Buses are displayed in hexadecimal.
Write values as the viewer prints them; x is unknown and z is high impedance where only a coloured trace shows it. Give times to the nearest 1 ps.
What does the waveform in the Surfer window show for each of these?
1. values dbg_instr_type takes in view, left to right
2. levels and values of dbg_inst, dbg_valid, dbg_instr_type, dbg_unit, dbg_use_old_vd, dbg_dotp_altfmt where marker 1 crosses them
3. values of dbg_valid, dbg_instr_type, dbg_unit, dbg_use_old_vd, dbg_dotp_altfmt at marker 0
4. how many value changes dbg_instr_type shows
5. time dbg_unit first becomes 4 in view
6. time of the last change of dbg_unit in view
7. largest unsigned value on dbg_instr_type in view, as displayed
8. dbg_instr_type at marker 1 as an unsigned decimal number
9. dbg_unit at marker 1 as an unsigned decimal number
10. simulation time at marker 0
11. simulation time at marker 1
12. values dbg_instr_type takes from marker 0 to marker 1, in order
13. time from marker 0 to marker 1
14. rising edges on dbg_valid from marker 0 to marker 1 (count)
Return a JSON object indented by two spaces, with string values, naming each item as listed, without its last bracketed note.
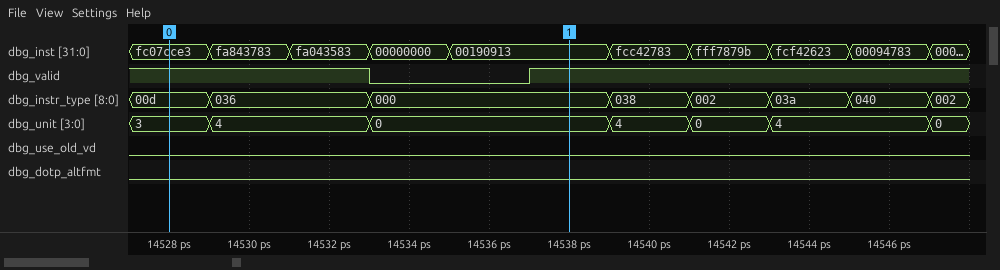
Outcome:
{
  "values dbg_instr_type takes in view, left to right": "00d, 036, 000, 038, 002, 03a, 040, 002",
  "levels and values of dbg_inst, dbg_valid, dbg_instr_type, dbg_unit, dbg_use_old_vd, dbg_dotp_altfmt where marker 1 crosses them": "dbg_inst=00190913, dbg_valid=1, dbg_instr_type=000, dbg_unit=0, dbg_use_old_vd=0, dbg_dotp_altfmt=0",
  "values of dbg_valid, dbg_instr_type, dbg_unit, dbg_use_old_vd, dbg_dotp_altfmt at marker 0": "dbg_valid=1, dbg_instr_type=00d, dbg_unit=3, dbg_use_old_vd=0, dbg_dotp_altfmt=0",
  "how many value changes dbg_instr_type shows": "7",
  "time dbg_unit first becomes 4 in view": "14529 ps",
  "time of the last change of dbg_unit in view": "14547 ps",
  "largest unsigned value on dbg_instr_type in view, as displayed": "040",
  "dbg_instr_type at marker 1 as an unsigned decimal number": "0",
  "dbg_unit at marker 1 as an unsigned decimal number": "0",
  "simulation time at marker 0": "14528 ps",
  "simulation time at marker 1": "14538 ps",
  "values dbg_instr_type takes from marker 0 to marker 1, in order": "00d, 036, 000",
  "time from marker 0 to marker 1": "10 ps",
  "rising edges on dbg_valid from marker 0 to marker 1": "1"
}
